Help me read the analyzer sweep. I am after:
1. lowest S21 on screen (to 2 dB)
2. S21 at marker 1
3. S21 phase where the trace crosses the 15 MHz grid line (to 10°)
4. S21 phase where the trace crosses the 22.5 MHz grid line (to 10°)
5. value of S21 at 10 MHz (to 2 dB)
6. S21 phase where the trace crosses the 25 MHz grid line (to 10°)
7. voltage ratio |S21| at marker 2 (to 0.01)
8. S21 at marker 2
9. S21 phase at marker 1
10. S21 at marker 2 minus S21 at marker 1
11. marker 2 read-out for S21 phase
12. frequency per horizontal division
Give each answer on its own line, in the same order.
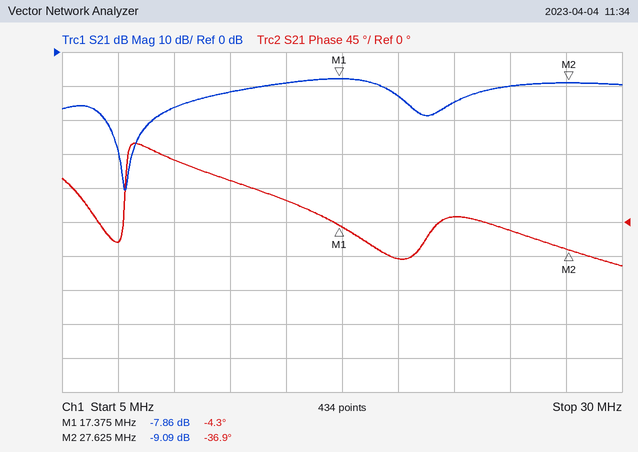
-40 dB
-7.86 dB
30°
10°
-16 dB
-10°
0.35
-9.09 dB
-4.3°
-1.23 dB
-36.9°
2.5 MHz
